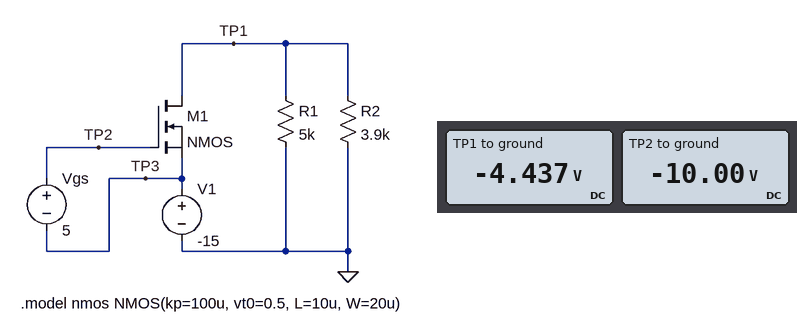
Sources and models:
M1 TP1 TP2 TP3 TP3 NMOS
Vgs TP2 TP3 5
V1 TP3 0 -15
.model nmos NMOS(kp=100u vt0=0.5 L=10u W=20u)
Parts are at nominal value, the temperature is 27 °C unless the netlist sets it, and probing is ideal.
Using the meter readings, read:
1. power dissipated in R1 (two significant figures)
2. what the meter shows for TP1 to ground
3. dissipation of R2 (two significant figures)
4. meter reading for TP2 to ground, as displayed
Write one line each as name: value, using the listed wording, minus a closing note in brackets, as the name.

power dissipated in R1: 3.9 mW
what the meter shows for TP1 to ground: -4.437 V
dissipation of R2: 5.0 mW
meter reading for TP2 to ground, as displayed: -10.00 V
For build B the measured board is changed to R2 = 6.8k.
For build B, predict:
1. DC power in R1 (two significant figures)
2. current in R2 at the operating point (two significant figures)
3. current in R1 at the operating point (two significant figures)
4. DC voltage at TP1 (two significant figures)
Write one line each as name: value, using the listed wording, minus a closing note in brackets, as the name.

DC power in R1: 6.8 mW
current in R2 at the operating point: 860 µA
current in R1 at the operating point: 1.2 mA
DC voltage at TP1: -5.8 V
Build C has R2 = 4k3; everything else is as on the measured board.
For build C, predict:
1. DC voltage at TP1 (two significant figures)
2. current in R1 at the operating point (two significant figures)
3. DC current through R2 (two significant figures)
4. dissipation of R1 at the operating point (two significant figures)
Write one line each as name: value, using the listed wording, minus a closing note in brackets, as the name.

DC voltage at TP1: -4.7 V
current in R1 at the operating point: 940 µA
DC current through R2: 1.1 mA
dissipation of R1 at the operating point: 4.4 mW
